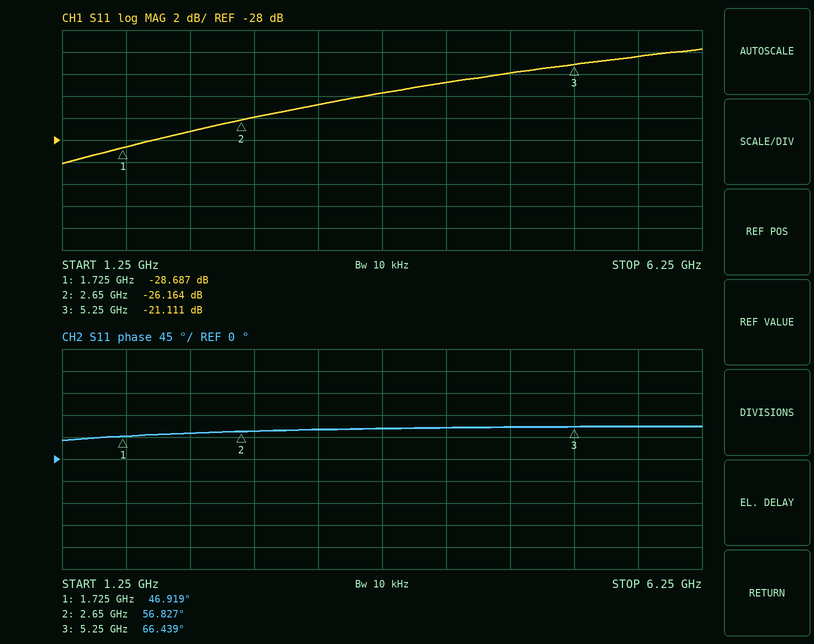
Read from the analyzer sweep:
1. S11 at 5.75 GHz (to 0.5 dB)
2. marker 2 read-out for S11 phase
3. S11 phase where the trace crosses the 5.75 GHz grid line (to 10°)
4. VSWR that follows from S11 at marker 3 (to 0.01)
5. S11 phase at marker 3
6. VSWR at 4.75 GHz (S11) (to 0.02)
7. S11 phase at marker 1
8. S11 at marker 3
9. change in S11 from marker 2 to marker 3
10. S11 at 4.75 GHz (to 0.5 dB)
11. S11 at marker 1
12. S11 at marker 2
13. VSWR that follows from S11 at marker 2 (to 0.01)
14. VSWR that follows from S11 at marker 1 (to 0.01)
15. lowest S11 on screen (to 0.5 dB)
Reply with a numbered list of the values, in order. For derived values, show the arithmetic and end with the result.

1. -20.5 dB
2. 56.827°
3. 70°
4. (1 + 0.0880)/(1 − 0.0880) ≈ 1.19
5. 66.439°
6. |Γ| = 10^(-22/20) = 0.0794; VSWR = (1 + 0.0794)/(1 − 0.0794) ≈ 1.17, so 1.18 to the nearest 0.02
7. 46.919°
8. -21.111 dB
9. -21.111 − (-26.164) = 5.053 dB
10. -22.0 dB
11. -28.687 dB
12. -26.164 dB
13. (1 + 0.0492)/(1 − 0.0492) ≈ 1.10
14. (1 + 0.0368)/(1 − 0.0368) ≈ 1.08
15. -30.0 dB
